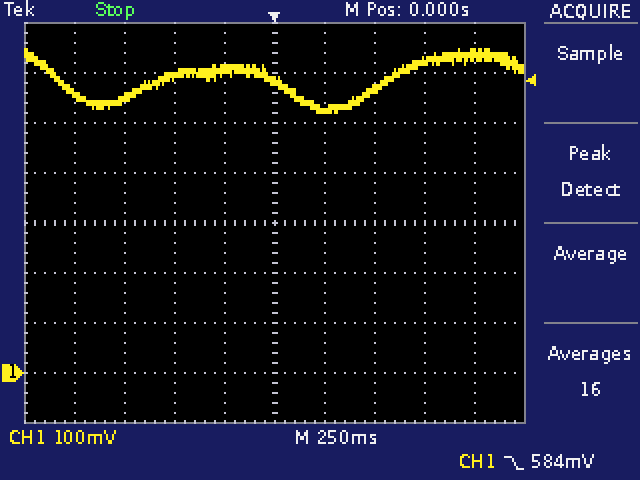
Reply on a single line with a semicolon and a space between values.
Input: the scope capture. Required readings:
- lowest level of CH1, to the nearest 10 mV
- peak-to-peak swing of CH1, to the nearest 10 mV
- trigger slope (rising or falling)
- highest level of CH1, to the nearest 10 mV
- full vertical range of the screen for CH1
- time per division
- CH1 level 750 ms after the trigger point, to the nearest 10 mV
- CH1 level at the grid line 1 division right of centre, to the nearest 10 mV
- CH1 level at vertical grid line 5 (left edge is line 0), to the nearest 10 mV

520 mV; 130 mV; falling; 650 mV; 800 mV; 250 ms; 620 mV; 520 mV; 580 mV
